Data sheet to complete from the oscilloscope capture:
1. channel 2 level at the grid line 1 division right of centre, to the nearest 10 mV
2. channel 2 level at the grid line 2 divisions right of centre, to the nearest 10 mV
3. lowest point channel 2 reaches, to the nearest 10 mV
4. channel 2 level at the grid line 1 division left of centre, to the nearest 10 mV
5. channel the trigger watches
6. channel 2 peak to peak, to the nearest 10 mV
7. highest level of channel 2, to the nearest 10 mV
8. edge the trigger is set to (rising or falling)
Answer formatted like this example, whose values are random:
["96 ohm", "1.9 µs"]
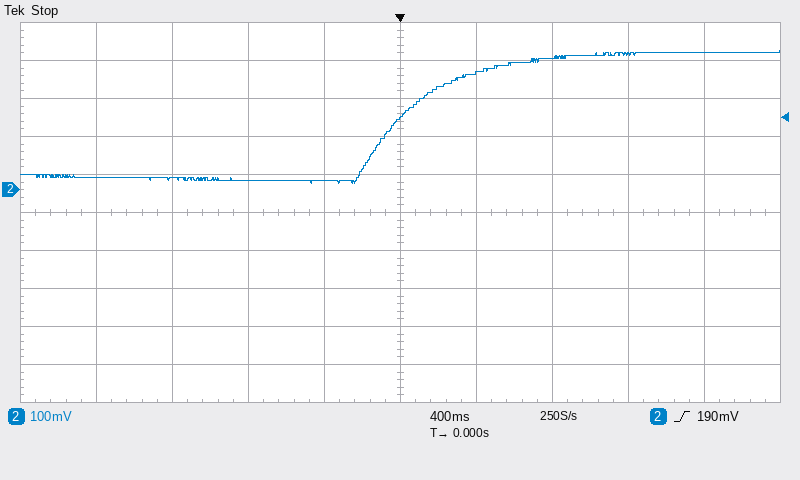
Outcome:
["310 mV", "350 mV", "20 mV", "20 mV", "channel 2", "350 mV", "370 mV", "rising"]
